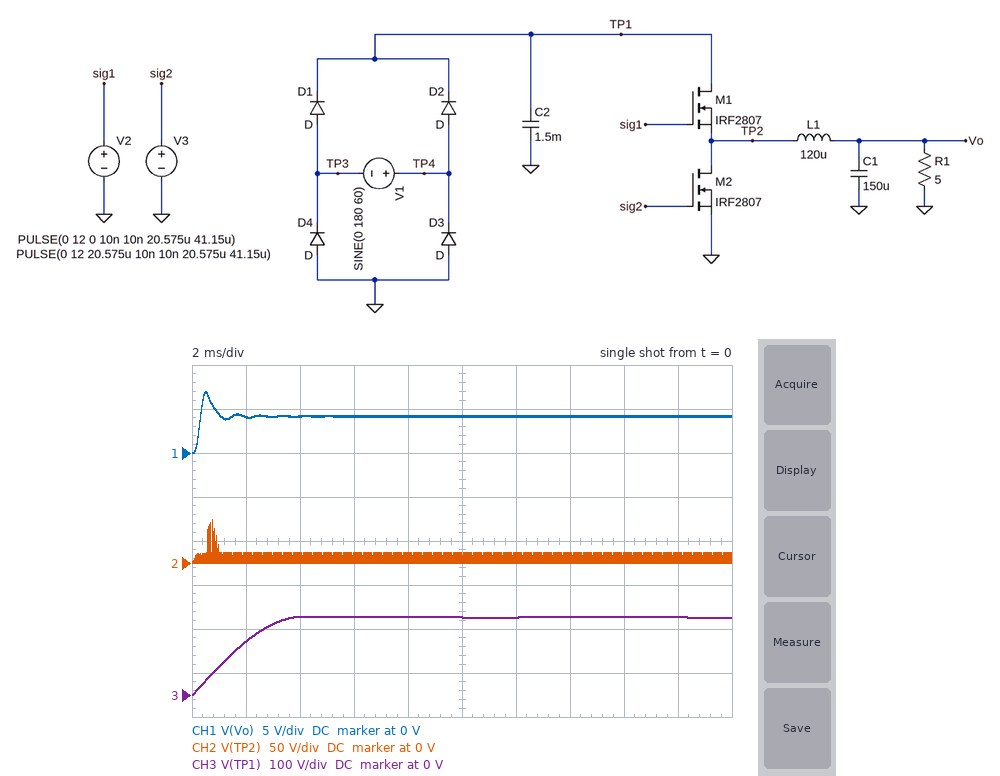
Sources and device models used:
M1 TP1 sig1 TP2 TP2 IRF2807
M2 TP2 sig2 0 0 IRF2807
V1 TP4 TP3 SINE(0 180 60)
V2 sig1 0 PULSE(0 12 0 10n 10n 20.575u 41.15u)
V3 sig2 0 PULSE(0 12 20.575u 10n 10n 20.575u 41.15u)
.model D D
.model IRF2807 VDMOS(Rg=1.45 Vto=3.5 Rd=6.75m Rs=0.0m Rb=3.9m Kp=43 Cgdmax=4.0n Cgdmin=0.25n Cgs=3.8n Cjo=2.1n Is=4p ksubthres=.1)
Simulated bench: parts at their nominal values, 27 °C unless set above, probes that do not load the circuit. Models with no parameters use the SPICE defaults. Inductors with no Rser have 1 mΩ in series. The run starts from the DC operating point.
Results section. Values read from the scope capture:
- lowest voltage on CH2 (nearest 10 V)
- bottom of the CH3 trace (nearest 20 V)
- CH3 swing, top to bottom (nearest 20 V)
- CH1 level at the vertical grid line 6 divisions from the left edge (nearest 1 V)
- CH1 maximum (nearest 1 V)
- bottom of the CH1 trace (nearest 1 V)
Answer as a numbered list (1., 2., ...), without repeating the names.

1. 0 V
2. 0 V
3. 180 V
4. 4 V
5. 7 V
6. 0 V
